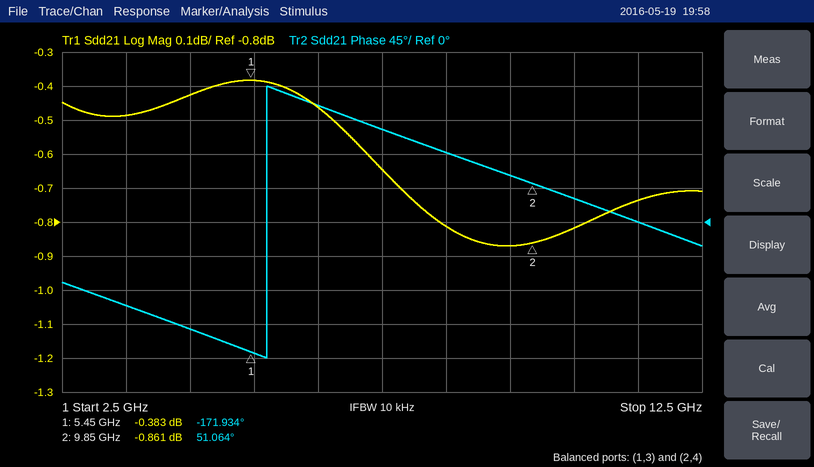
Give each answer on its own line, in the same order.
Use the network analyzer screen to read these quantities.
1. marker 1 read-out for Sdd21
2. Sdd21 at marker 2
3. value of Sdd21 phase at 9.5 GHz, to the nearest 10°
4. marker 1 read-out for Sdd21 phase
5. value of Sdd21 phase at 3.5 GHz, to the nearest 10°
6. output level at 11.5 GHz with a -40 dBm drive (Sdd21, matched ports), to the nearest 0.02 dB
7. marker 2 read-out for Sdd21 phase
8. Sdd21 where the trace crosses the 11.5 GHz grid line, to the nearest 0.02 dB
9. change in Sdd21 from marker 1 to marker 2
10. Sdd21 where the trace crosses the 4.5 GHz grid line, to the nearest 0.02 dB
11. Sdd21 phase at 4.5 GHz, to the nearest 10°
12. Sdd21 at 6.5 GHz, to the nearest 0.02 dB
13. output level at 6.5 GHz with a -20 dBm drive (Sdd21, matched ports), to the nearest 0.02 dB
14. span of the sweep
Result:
-0.383 dB
-0.861 dB
60°
-171.934°
-110°
-40.74 dBm
51.064°
-0.74 dB
-0.478 dB
-0.42 dB
-140°
-0.46 dB
-20.46 dBm
10 GHz
